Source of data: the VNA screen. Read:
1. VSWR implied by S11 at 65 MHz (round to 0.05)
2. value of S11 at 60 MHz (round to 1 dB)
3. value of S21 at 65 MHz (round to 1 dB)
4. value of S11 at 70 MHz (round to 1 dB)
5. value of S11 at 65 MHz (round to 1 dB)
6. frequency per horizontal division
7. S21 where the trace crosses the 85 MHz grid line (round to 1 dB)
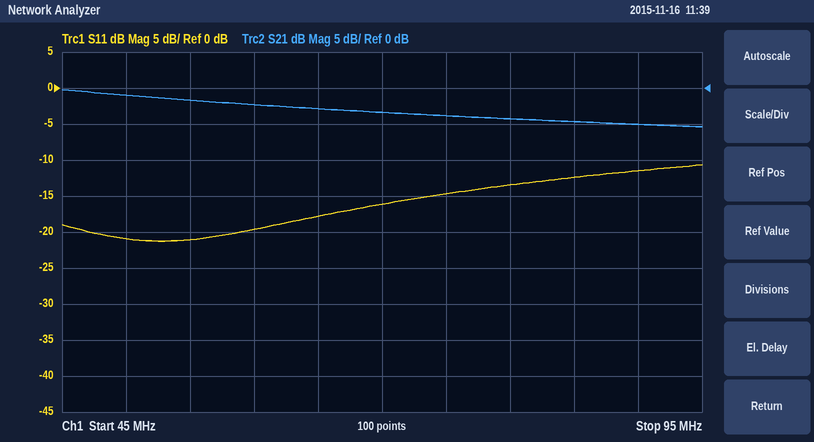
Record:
1.30
-20 dB
-3 dB
-16 dB
-18 dB
5 MHz
-5 dB
